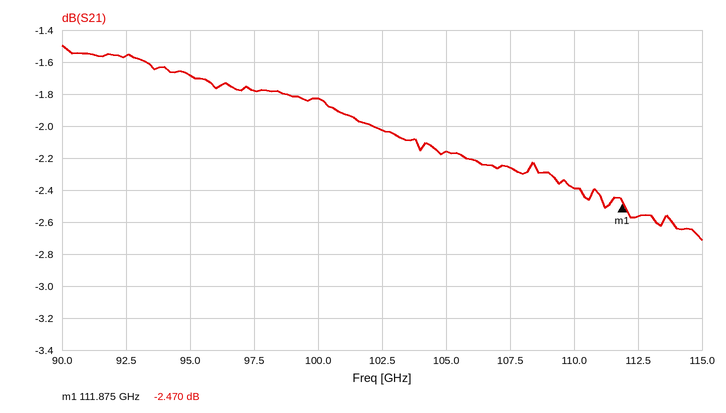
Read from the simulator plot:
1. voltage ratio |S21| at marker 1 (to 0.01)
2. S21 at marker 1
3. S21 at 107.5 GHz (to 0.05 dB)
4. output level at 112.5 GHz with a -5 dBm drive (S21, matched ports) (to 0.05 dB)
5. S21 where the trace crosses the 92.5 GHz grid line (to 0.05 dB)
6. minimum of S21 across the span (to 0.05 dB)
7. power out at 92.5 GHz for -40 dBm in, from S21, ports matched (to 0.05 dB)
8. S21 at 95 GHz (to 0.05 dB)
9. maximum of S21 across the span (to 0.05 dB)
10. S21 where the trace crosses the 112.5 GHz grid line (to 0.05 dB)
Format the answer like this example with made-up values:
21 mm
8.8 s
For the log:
0.75
-2.470 dB
-2.25 dB
-7.55 dBm
-1.55 dB
-2.70 dB
-41.55 dBm
-1.70 dB
-1.50 dB
-2.55 dB
